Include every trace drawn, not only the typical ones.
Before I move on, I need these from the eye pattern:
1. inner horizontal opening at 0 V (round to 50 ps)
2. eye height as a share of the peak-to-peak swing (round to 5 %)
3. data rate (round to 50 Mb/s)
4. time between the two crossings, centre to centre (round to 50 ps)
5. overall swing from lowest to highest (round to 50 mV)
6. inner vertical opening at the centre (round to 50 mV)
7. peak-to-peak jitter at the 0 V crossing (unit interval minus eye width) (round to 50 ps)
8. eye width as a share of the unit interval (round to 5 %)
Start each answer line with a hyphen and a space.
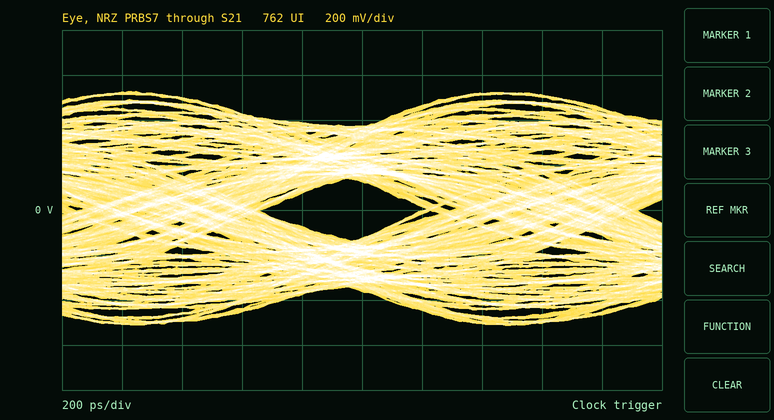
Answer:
- 550 ps
- 25 %
- 800 Mb/s
- 1.25 ns
- 1.05 V
- 250 mV
- 700 ps
- 45 %
